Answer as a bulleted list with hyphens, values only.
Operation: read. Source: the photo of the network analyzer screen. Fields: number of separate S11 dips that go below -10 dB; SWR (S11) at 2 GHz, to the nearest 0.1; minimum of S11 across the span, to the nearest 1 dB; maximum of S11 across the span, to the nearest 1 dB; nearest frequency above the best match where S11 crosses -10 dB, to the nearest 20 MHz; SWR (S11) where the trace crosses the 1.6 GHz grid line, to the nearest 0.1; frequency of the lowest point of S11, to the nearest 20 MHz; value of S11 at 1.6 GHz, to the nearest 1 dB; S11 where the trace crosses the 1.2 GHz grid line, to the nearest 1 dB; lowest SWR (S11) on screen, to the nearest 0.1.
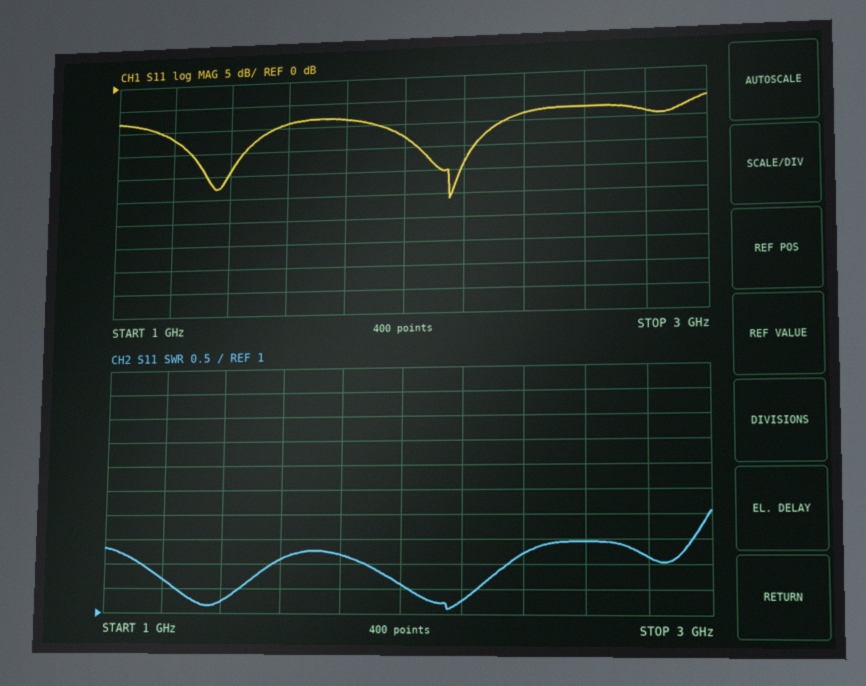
- 2
- 1.6
- -26 dB
- -6 dB
- 2.34 GHz
- 2.1
- 2.16 GHz
- -9 dB
- -12 dB
- 1.1
